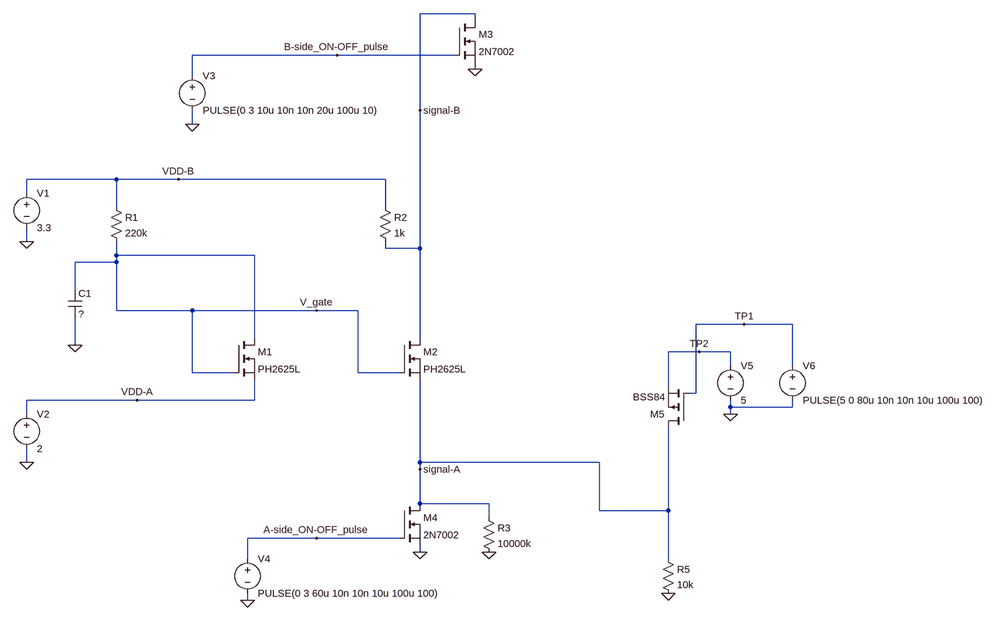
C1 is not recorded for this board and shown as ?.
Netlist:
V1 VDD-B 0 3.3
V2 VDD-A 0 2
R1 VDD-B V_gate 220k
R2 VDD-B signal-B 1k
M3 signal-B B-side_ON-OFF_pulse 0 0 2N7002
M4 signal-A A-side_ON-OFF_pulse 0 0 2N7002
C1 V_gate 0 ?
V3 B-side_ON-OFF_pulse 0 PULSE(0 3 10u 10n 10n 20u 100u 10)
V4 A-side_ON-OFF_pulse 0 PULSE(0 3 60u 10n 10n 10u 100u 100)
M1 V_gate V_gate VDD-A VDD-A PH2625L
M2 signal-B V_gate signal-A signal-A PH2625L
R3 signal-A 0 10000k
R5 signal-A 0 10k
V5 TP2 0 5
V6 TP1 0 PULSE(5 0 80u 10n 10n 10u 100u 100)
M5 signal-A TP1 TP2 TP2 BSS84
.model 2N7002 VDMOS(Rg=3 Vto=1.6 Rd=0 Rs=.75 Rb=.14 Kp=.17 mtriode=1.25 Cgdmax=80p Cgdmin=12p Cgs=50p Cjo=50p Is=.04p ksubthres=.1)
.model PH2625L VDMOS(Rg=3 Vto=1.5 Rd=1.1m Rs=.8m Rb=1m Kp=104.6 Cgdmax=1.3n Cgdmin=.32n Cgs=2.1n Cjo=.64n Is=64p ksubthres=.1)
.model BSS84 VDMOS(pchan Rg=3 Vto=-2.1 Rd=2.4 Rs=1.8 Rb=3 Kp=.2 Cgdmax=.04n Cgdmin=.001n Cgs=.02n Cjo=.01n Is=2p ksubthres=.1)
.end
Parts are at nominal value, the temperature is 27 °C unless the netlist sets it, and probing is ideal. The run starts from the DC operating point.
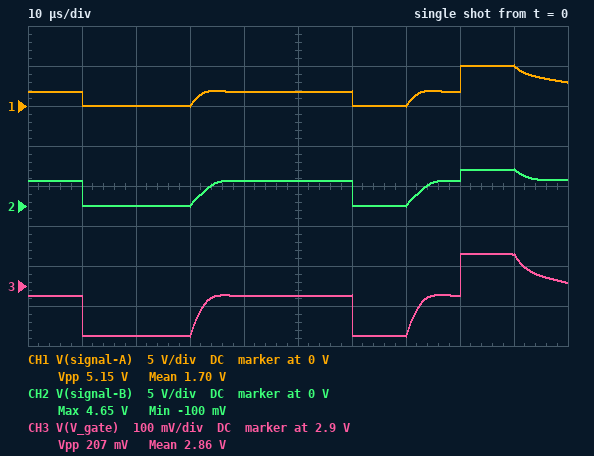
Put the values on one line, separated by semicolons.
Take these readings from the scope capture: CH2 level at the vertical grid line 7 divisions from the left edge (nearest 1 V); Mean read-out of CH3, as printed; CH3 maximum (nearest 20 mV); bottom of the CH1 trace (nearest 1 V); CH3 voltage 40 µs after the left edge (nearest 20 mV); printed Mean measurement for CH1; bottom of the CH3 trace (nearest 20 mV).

0 V; 2.86 V; 2.98 V; 0 V; 2.88 V; 1.70 V; 2.78 V
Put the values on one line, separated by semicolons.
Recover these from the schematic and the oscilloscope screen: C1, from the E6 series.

68 nF
